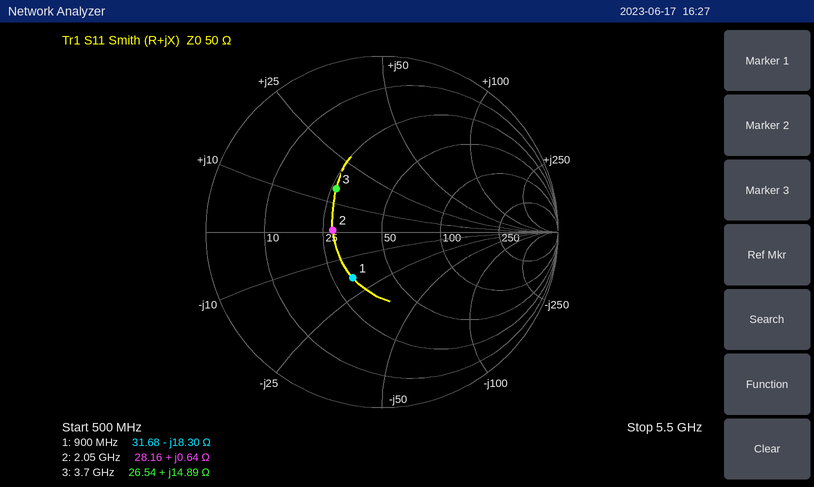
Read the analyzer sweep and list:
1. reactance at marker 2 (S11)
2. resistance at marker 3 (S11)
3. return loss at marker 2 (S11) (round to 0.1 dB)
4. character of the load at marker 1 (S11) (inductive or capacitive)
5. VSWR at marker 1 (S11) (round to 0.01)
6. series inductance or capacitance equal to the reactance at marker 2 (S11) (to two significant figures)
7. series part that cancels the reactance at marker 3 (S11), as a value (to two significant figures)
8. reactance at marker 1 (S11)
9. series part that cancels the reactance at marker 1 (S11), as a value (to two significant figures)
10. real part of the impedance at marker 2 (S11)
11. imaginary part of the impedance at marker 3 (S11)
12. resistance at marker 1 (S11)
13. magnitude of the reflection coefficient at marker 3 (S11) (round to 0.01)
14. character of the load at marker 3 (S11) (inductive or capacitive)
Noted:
+0.64 Ω
26.54 Ω
11.1 dB
capacitive
1.90
50 pH
2.9 pF
-18.30 Ω
3.2 nH
28.16 Ω
+14.89 Ω
31.68 Ω
0.36
inductive
